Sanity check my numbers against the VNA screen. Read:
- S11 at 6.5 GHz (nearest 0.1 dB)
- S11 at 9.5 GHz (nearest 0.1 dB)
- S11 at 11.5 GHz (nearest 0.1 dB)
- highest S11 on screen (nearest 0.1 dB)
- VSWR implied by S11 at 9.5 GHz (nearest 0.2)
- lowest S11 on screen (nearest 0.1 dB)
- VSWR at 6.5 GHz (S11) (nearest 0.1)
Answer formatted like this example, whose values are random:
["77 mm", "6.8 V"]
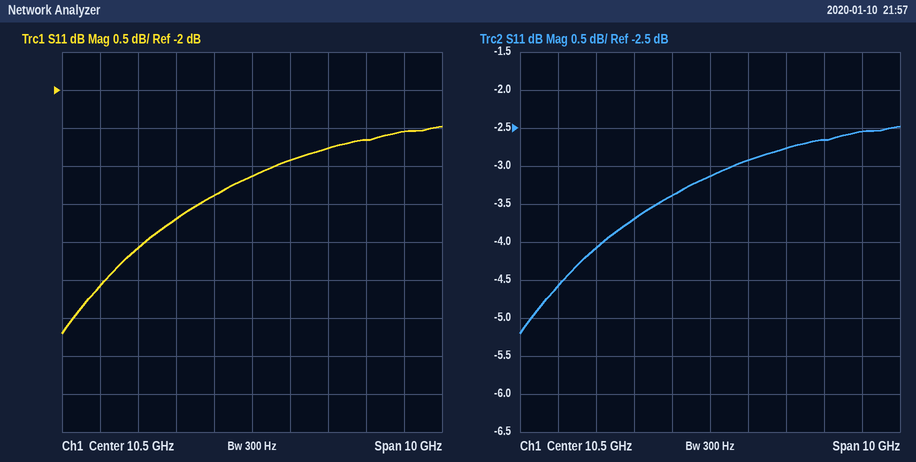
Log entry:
["-4.6 dB", "-3.4 dB", "-2.9 dB", "-2.5 dB", "5.2", "-5.2 dB", "3.9"]
